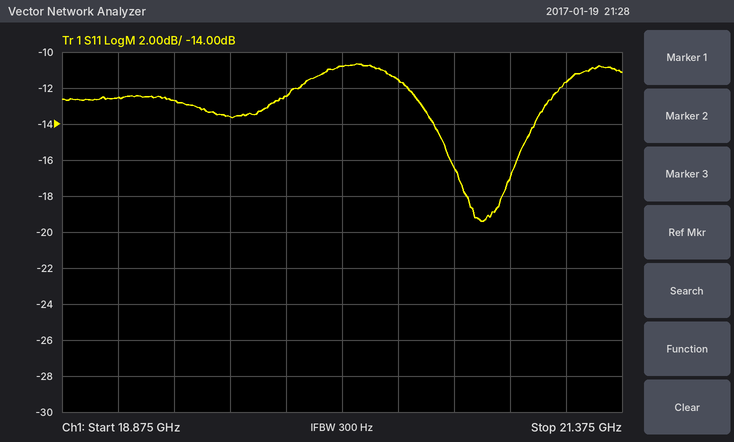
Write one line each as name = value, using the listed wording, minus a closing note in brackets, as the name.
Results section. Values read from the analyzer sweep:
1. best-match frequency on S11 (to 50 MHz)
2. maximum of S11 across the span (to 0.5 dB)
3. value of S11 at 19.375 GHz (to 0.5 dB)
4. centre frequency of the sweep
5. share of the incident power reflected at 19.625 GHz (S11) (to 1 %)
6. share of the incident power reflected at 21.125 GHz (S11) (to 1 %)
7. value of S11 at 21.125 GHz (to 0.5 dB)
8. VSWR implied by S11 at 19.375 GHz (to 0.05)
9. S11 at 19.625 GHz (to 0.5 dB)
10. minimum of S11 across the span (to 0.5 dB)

best-match frequency on S11 = 20.75 GHz
maximum of S11 across the span = -10.5 dB
value of S11 at 19.375 GHz = -12.5 dB
centre frequency of the sweep = 20.125 GHz
share of the incident power reflected at 19.625 GHz (S11) = 4 %
share of the incident power reflected at 21.125 GHz (S11) = 7 %
value of S11 at 21.125 GHz = -11.5 dB
VSWR implied by S11 at 19.375 GHz = 1.60
S11 at 19.625 GHz = -13.5 dB
minimum of S11 across the span = -19.5 dB
